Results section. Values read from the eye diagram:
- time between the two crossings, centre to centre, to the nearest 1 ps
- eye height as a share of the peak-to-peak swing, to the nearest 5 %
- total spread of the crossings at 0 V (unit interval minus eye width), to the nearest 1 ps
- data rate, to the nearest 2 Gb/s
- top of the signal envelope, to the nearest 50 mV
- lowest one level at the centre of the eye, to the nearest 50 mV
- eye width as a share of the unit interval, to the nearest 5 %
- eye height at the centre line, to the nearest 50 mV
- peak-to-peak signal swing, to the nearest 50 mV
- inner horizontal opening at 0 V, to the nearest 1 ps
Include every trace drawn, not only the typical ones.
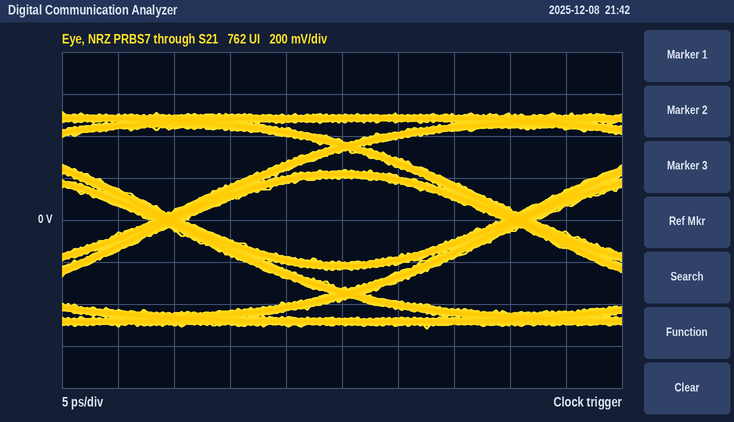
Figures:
31 ps
40 %
3 ps
32 Gb/s
500 mV
200 mV
90 %
400 mV
1.05 V
28 ps
